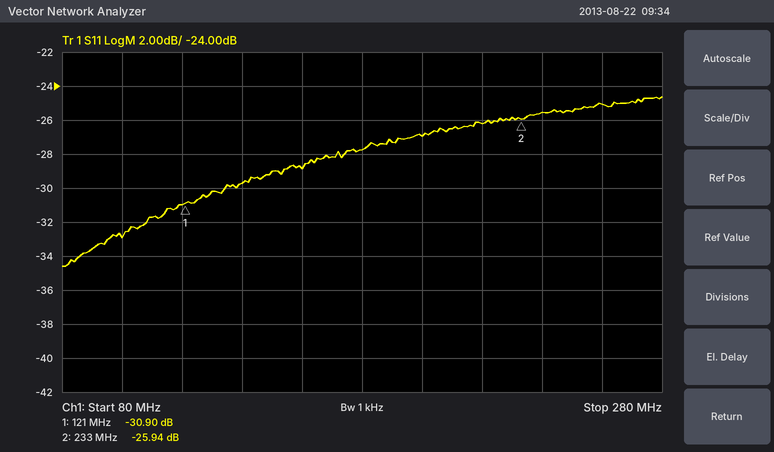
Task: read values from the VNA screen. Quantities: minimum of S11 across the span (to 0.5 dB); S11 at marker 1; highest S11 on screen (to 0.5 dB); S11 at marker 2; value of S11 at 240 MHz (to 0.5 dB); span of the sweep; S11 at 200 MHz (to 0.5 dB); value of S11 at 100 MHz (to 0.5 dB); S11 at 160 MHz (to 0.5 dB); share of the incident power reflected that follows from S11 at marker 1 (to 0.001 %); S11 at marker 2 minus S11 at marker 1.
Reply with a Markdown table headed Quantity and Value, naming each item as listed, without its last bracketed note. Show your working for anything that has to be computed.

| Quantity | Value |
|---|---|
| minimum of S11 across the span | -34.5 dB |
| S11 at marker 1 | -30.90 dB |
| highest S11 on screen | -24.5 dB |
| S11 at marker 2 | -25.94 dB |
| value of S11 at 240 MHz | -25.5 dB |
| span of the sweep | 200 MHz |
| S11 at 200 MHz | -27.0 dB |
| value of S11 at 100 MHz | -33.0 dB |
| S11 at 160 MHz | -29.0 dB |
| share of the incident power reflected that follows from S11 at marker 1 | 10^(-30.9/10) ≈ 0.081 % |
| S11 at marker 2 minus S11 at marker 1 | -25.94 − (-30.9) = 4.96 dB |
